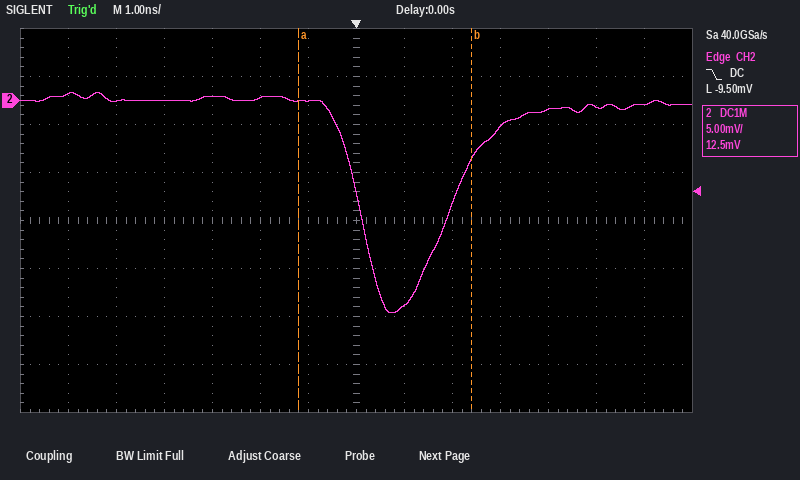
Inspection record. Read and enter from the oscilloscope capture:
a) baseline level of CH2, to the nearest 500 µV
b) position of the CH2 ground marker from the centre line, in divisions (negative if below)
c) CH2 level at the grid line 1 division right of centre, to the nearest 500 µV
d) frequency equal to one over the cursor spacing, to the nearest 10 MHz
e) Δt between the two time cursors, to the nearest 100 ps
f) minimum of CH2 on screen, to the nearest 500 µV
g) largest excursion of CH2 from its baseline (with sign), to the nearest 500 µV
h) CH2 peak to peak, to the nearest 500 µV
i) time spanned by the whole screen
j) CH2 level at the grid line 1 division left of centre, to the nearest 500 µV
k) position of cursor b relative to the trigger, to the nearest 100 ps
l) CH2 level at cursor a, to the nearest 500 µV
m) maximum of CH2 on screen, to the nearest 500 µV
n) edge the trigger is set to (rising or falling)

0.0 mV
+2.5 div
-21.5 mV
280 MHz
3.6 ns
-22.0 mV
-22.0 mV
23.0 mV
14 ns
0.0 mV
+2.4 ns
0.0 mV
1.0 mV
falling
